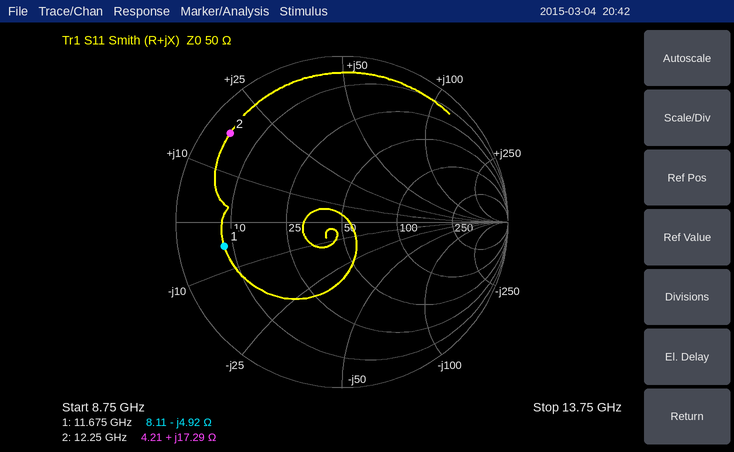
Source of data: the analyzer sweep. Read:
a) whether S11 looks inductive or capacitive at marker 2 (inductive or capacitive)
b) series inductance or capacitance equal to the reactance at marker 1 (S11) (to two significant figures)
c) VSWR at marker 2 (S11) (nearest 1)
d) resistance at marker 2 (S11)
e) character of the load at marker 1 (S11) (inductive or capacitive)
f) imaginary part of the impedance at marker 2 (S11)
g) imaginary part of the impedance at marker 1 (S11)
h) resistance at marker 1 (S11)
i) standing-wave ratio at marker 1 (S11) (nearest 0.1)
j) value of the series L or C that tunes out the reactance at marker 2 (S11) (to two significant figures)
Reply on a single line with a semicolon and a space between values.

inductive; 2.8 pF; 13; 4.21 Ω; capacitive; +17.29 Ω; -4.92 Ω; 8.11 Ω; 6.2; 750 fF
